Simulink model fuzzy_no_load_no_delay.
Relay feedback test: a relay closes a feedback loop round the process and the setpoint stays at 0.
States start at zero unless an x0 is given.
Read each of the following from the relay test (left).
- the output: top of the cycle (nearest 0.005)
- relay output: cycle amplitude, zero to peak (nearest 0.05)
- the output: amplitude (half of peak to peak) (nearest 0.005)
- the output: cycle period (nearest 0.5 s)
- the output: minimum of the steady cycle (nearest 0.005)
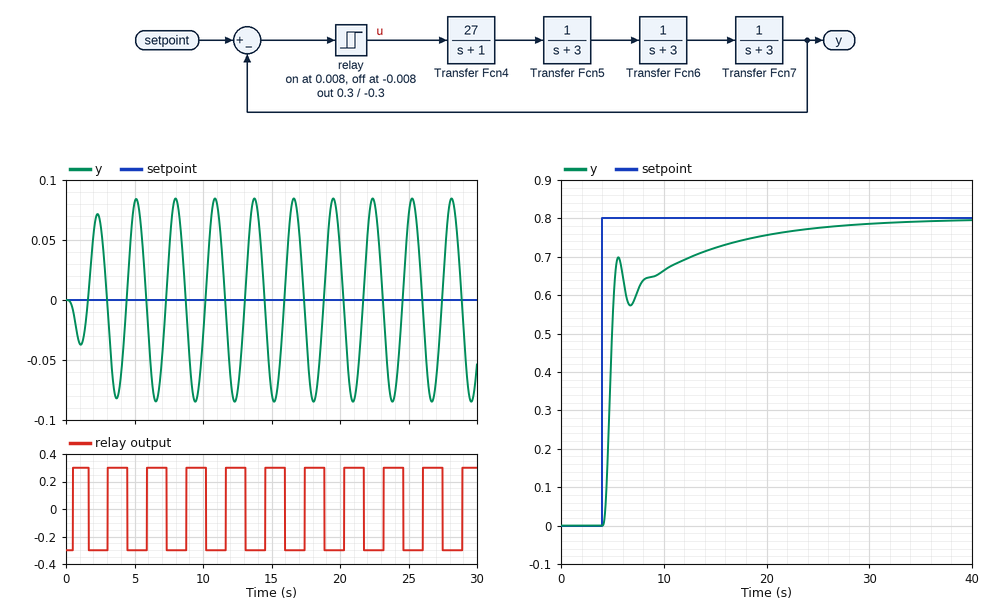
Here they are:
0.085
0.30
0.085
3.0 s
-0.085
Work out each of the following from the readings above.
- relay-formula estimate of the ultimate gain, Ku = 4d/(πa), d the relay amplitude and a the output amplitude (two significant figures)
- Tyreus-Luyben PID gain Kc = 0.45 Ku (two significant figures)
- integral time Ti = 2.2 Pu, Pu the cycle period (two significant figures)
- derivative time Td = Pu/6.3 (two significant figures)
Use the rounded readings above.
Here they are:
4.5
2.0
6.6 s
0.48 s
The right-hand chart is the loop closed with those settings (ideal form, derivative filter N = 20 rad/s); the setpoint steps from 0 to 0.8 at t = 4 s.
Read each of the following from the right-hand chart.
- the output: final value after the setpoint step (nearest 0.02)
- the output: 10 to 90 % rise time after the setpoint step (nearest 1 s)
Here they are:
0.80
10 s
